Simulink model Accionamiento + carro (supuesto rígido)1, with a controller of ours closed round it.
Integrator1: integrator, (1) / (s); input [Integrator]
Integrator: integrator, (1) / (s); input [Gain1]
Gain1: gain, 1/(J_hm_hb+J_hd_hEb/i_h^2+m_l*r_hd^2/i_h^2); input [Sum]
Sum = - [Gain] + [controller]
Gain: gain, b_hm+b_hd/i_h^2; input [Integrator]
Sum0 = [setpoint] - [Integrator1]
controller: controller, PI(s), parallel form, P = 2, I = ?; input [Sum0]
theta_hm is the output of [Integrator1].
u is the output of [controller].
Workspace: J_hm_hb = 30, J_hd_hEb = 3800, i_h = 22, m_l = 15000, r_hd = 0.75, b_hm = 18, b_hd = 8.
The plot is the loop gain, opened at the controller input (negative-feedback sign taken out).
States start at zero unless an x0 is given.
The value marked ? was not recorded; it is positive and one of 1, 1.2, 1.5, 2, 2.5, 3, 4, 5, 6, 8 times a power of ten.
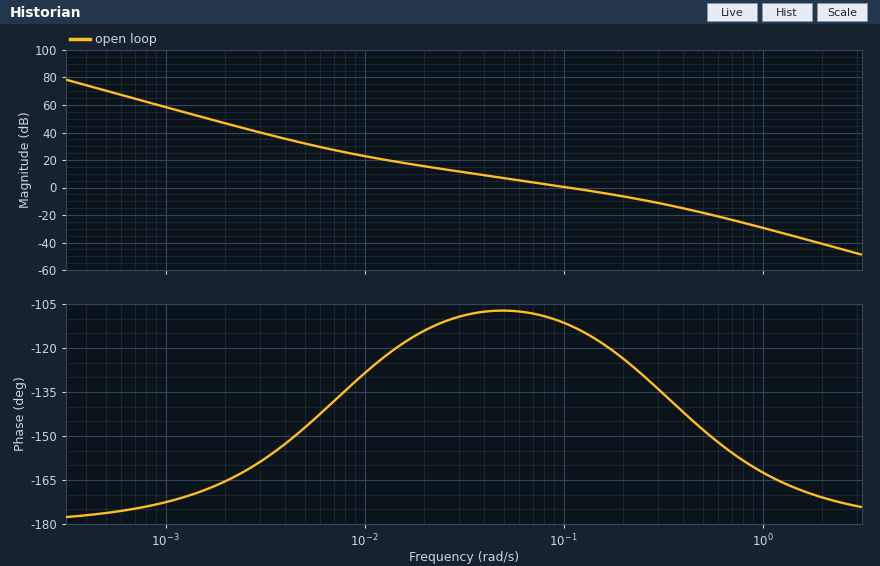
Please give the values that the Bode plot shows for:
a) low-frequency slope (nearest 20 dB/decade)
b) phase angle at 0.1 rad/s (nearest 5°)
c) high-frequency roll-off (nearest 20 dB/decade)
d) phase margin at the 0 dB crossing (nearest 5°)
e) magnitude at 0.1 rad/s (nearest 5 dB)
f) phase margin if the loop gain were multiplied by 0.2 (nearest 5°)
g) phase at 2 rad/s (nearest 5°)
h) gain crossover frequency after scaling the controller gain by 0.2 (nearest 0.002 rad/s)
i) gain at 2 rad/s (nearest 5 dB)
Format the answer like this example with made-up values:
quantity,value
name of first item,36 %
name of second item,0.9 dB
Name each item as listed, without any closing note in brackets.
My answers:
quantity,value
low-frequency slope,-40 dB/decade
phase angle at 0.1 rad/s,-110°
high-frequency roll-off,-40 dB/decade
phase margin at the 0 dB crossing,70°
magnitude at 0.1 rad/s,0 dB
phase margin if the loop gain were multiplied by 0.2,70°
phase at 2 rad/s,-170°
gain crossover frequency after scaling the controller gain by 0.2,0.024 rad/s
gain at 2 rad/s,-40 dB
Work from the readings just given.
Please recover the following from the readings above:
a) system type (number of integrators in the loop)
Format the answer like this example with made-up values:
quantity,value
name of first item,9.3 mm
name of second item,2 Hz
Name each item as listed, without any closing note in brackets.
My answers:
quantity,value
system type,2
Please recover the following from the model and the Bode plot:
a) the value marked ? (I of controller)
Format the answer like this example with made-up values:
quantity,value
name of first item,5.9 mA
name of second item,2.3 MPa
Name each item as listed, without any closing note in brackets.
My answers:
quantity,value
the value marked ?,0.015
